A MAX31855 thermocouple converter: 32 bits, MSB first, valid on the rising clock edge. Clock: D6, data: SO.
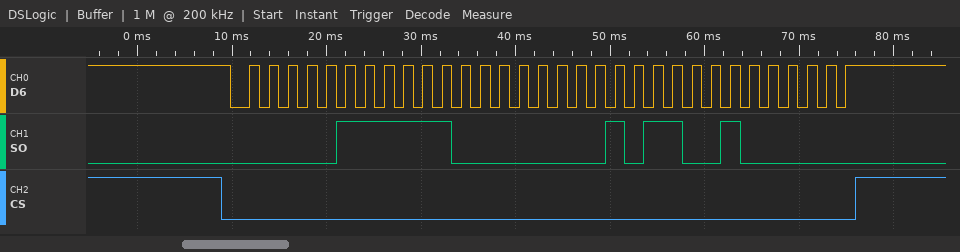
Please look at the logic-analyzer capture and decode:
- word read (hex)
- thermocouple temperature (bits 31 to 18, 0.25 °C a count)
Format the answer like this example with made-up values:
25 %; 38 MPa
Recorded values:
0x07E01640; 126.00 °C
